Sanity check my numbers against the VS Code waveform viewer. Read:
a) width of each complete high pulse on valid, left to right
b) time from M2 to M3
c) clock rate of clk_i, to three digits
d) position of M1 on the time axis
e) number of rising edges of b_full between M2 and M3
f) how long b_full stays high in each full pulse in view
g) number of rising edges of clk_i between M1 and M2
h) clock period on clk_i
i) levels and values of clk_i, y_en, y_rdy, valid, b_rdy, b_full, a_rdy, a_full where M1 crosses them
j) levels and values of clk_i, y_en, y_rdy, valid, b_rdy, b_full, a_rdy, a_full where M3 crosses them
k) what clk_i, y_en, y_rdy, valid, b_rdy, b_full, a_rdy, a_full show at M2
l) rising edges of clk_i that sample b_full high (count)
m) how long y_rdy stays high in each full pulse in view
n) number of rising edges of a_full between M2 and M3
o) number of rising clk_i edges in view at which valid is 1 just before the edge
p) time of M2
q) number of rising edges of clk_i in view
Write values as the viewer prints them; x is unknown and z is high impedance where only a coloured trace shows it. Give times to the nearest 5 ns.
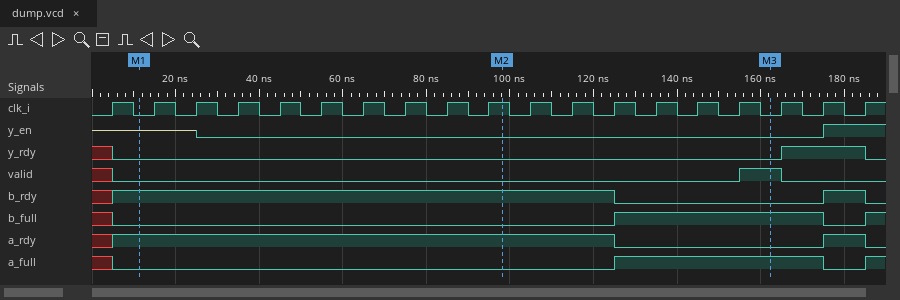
10 ns
65 ns
100 MHz
10 ns
1
50 ns
9
10 ns
clk_i=0, y_en=z, y_rdy=0, valid=0, b_rdy=1, b_full=0, a_rdy=1, a_full=0
clk_i=0, y_en=0, y_rdy=0, valid=1, b_rdy=0, b_full=1, a_rdy=0, a_full=1
clk_i=1, y_en=0, y_rdy=0, valid=0, b_rdy=1, b_full=0, a_rdy=1, a_full=0
5
20 ns
1
1
100 ns
19
